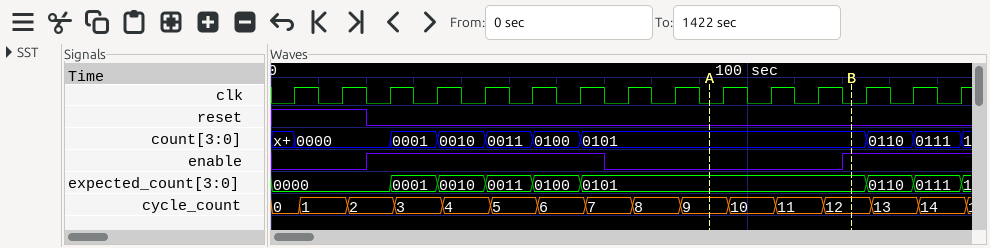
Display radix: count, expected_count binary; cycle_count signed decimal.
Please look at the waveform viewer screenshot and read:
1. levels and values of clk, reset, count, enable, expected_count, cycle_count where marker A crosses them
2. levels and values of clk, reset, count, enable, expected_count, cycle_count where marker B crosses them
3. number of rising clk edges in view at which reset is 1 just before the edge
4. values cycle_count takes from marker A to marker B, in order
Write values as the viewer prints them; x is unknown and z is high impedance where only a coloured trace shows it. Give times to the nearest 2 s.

clk=0, reset=0, count=0101, enable=0, expected_count=0101, cycle_count=9
clk=0, reset=0, count=0101, enable=1, expected_count=0101, cycle_count=12
2
9, 10, 11, 12
